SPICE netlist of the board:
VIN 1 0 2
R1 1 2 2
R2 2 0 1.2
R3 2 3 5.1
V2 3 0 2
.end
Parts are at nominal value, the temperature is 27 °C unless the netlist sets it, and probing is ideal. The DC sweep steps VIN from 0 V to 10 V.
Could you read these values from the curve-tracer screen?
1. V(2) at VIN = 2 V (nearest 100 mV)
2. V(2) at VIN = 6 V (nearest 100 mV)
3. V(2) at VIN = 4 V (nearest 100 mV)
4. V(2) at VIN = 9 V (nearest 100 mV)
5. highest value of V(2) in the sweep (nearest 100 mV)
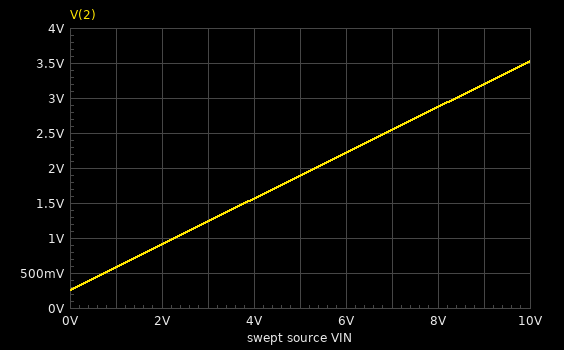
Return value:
900 mV
2.2 V
1.6 V
3.2 V
3.5 V
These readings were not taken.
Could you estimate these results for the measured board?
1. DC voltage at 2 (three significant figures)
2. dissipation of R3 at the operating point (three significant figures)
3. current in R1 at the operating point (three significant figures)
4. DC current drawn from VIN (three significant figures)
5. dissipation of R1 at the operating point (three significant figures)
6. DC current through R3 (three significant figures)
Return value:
910 mV
233 mW
545 mA
545 mA
594 mW
214 mA
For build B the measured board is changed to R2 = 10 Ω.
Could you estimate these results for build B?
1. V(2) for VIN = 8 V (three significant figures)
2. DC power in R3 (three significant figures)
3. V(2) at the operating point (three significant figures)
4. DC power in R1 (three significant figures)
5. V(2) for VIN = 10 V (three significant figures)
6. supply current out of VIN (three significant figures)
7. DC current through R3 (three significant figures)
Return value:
5.52 V
12.4 mW
1.75 V
31.6 mW
6.77 V
126 mA
49.3 mA
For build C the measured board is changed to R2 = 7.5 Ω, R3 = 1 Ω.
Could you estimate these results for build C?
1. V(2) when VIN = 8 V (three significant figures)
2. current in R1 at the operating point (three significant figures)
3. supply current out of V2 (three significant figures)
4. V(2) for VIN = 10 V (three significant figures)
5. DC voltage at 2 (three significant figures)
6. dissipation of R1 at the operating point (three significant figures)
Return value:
3.67 V
81.6 mA
163 mA
4.29 V
1.84 V
13.3 mW
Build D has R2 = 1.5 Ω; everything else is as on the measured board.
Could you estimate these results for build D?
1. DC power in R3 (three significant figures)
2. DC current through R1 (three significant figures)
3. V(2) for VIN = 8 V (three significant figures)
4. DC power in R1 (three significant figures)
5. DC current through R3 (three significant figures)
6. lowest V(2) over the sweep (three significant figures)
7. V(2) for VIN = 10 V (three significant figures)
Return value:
188 mW
489 mA
3.22 V
479 mW
192 mA
288 mV
3.96 V
